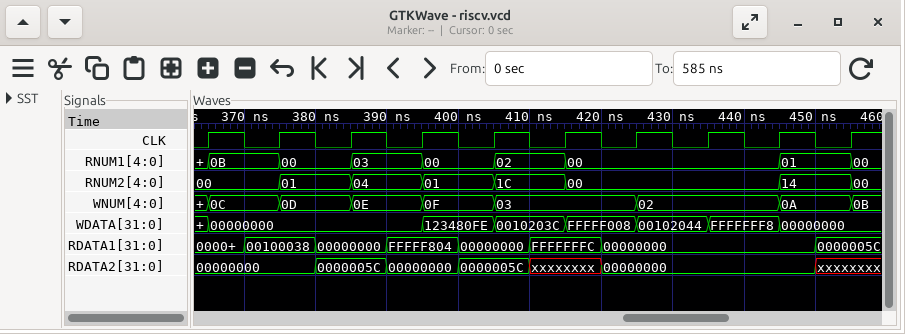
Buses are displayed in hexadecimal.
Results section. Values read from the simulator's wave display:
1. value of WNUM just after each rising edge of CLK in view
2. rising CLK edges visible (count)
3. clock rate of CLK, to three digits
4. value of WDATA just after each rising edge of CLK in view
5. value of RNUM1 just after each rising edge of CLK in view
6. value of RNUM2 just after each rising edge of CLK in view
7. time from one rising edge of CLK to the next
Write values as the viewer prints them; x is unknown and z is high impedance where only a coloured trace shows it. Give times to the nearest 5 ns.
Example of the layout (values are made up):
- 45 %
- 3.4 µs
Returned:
- 0C, 0D, 0E, 0F, 03, 03, 02, 02, 0A, 0B
- 10
- 100 MHz
- 00000000, 00000000, 00000000, 123480FE, 0010203C, FFFFF008, 00102044, FFFFFFF8, 00000000, 00000000
- 0B, 00, 03, 00, 02, 00, 00, 00, 01, 00
- 00, 01, 04, 01, 1C, 00, 00, 00, 14, 00
- 10 ns
